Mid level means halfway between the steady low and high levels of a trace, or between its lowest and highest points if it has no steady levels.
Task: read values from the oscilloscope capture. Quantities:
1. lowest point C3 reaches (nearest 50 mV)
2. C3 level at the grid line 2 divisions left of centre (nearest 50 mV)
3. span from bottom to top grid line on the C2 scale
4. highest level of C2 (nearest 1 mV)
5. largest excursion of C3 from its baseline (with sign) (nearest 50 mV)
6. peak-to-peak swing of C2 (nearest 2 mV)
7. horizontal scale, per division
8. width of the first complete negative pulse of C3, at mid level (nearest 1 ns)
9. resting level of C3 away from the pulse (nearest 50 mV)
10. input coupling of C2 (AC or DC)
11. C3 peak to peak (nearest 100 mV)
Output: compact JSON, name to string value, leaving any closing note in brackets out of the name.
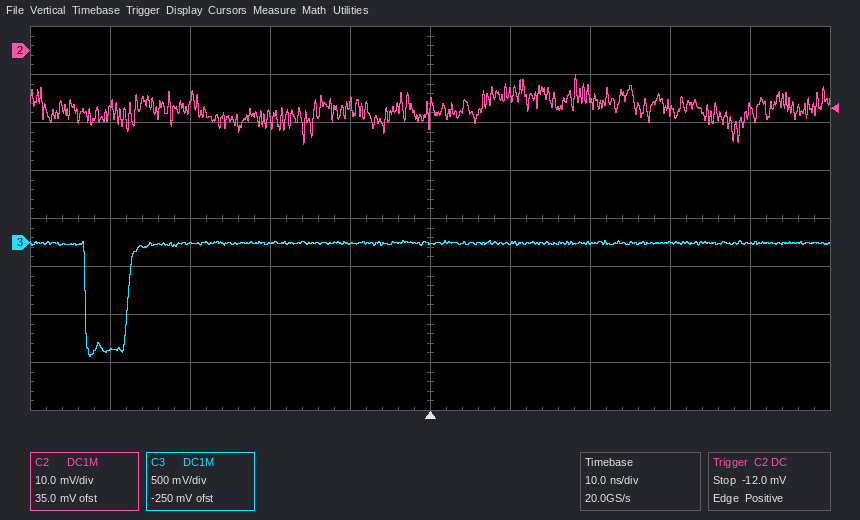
{"lowest point C3 reaches": "-1.20 V", "C3 level at the grid line 2 divisions left of centre": "0 mV", "span from bottom to top grid line on the C2 scale": "80 mV", "highest level of C2": "-5 mV", "largest excursion of C3 from its baseline (with sign)": "-1.20 V", "peak-to-peak swing of C2": "14 mV", "horizontal scale, per division": "10 ns", "width of the first complete negative pulse of C3, at mid level": "5 ns", "resting level of C3 away from the pulse": "0 mV", "input coupling of C2": "DC", "C3 peak to peak": "1.20 V"}
